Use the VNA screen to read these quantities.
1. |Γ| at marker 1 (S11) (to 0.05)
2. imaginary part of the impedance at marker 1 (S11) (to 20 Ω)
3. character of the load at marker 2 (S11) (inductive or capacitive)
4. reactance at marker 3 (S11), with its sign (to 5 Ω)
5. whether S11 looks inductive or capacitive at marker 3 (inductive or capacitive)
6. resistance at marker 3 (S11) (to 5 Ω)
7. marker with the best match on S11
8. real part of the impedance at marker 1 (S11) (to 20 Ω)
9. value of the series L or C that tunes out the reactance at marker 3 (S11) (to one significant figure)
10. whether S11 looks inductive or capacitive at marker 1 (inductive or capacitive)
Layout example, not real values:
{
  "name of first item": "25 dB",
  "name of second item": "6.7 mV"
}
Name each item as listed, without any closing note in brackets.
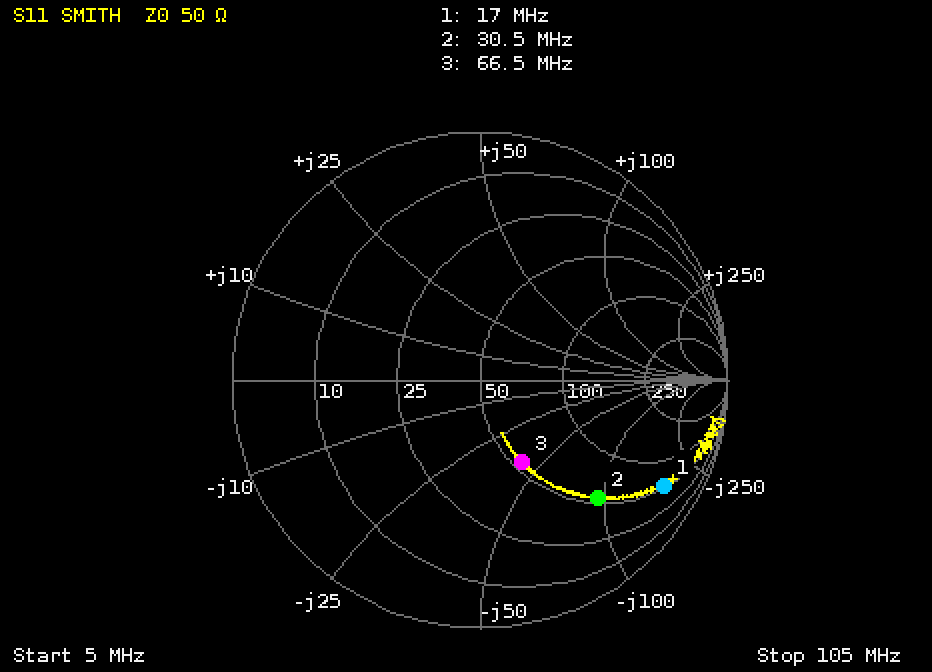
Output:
{
  "|Γ| at marker 1 (S11)": "0.85",
  "imaginary part of the impedance at marker 1 (S11)": "-180 Ω",
  "character of the load at marker 2 (S11)": "capacitive",
  "reactance at marker 3 (S11), with its sign": "-40 Ω",
  "whether S11 looks inductive or capacitive at marker 3": "capacitive",
  "resistance at marker 3 (S11)": "55 Ω",
  "marker with the best match on S11": "marker 3",
  "real part of the impedance at marker 1 (S11)": "60 Ω",
  "value of the series L or C that tunes out the reactance at marker 3 (S11)": "100 nH",
  "whether S11 looks inductive or capacitive at marker 1": "capacitive"
}
